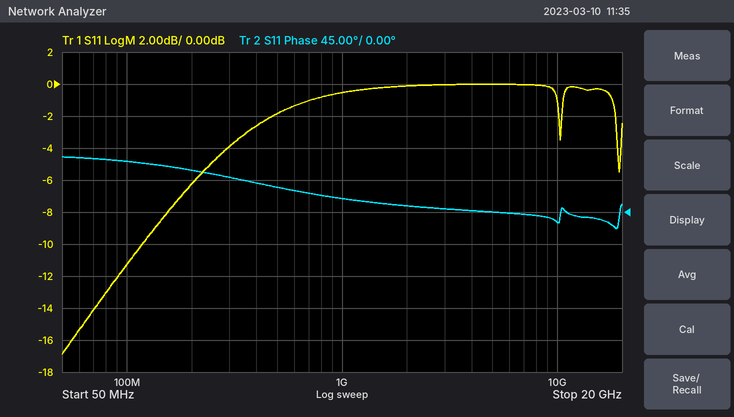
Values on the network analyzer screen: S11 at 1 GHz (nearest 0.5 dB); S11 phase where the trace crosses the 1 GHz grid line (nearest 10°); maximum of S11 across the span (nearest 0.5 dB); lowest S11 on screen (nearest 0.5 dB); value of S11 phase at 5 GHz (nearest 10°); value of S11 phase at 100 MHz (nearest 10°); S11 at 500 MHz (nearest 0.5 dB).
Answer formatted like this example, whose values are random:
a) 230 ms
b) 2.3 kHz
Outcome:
a) -0.5 dB
b) 20°
c) 0.0 dB
d) -17.0 dB
e) 0°
f) 70°
g) -2.0 dB
